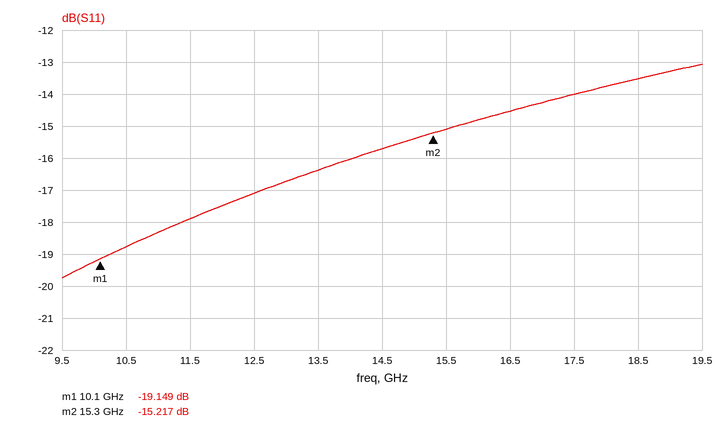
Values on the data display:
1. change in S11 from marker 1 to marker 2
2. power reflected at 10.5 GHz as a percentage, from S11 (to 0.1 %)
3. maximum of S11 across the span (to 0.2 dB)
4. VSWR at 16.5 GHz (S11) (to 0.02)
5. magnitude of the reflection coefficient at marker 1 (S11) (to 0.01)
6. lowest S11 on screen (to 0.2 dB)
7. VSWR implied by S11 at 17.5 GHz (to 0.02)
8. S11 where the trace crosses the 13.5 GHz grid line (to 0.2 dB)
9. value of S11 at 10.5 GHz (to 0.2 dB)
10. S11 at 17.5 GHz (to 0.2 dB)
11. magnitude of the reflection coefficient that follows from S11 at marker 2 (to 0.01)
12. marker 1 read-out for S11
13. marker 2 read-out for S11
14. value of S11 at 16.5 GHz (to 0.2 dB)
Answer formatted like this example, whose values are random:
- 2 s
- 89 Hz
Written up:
- 3.932 dB
- 1.3 %
- -13.0 dB
- 1.46
- 0.11
- -19.8 dB
- 1.50
- -16.4 dB
- -18.8 dB
- -14.0 dB
- 0.17
- -19.149 dB
- -15.217 dB
- -14.6 dB
